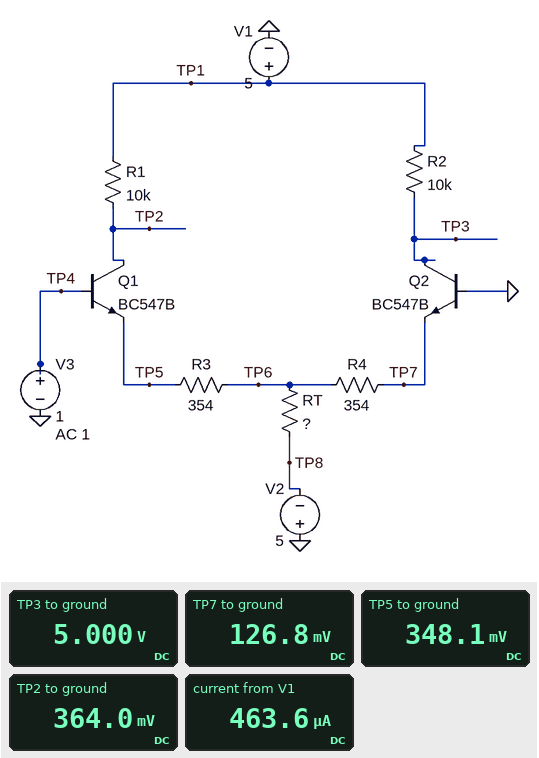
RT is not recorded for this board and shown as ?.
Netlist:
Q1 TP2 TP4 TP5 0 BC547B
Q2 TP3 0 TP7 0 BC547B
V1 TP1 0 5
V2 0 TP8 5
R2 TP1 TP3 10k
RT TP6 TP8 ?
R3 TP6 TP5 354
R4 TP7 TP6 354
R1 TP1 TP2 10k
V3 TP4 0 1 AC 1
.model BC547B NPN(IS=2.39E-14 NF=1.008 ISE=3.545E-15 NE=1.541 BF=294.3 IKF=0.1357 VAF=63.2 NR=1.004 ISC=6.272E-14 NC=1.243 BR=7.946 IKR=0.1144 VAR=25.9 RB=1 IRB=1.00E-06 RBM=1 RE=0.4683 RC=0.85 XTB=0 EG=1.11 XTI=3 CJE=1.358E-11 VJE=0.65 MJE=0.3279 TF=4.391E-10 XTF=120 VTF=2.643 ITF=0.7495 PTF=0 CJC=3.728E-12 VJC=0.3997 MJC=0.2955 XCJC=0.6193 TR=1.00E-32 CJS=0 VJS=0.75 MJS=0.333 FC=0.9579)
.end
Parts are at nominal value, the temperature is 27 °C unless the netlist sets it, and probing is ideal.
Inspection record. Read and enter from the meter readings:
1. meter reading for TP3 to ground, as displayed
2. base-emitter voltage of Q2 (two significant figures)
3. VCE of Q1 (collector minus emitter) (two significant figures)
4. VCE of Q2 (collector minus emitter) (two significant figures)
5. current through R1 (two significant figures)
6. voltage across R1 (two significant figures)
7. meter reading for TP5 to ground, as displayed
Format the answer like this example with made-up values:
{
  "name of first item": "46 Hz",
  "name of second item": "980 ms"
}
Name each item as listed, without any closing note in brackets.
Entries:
{
  "meter reading for TP3 to ground, as displayed": "5.000 V",
  "base-emitter voltage of Q2": "-130 mV",
  "VCE of Q1 (collector minus emitter)": "16 mV",
  "VCE of Q2 (collector minus emitter)": "4.9 V",
  "current through R1": "460 µA",
  "voltage across R1": "4.6 V",
  "meter reading for TP5 to ground, as displayed": "348.1 mV"
}
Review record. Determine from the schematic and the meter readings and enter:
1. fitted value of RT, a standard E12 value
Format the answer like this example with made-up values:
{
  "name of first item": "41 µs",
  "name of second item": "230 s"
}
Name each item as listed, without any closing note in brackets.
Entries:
{
  "fitted value of RT, a standard E12 value": "8.2 kΩ"
}
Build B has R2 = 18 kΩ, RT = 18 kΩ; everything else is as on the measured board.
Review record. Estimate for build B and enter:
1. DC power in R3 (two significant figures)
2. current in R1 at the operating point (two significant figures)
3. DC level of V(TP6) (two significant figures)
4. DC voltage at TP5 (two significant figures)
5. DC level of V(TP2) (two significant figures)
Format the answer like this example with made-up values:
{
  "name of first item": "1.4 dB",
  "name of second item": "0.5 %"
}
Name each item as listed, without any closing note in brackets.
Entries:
{
  "DC power in R3": "31 µW",
  "current in R1 at the operating point": "290 µA",
  "DC level of V(TP6)": "290 mV",
  "DC voltage at TP5": "390 mV",
  "DC level of V(TP2)": "2.1 V"
}
